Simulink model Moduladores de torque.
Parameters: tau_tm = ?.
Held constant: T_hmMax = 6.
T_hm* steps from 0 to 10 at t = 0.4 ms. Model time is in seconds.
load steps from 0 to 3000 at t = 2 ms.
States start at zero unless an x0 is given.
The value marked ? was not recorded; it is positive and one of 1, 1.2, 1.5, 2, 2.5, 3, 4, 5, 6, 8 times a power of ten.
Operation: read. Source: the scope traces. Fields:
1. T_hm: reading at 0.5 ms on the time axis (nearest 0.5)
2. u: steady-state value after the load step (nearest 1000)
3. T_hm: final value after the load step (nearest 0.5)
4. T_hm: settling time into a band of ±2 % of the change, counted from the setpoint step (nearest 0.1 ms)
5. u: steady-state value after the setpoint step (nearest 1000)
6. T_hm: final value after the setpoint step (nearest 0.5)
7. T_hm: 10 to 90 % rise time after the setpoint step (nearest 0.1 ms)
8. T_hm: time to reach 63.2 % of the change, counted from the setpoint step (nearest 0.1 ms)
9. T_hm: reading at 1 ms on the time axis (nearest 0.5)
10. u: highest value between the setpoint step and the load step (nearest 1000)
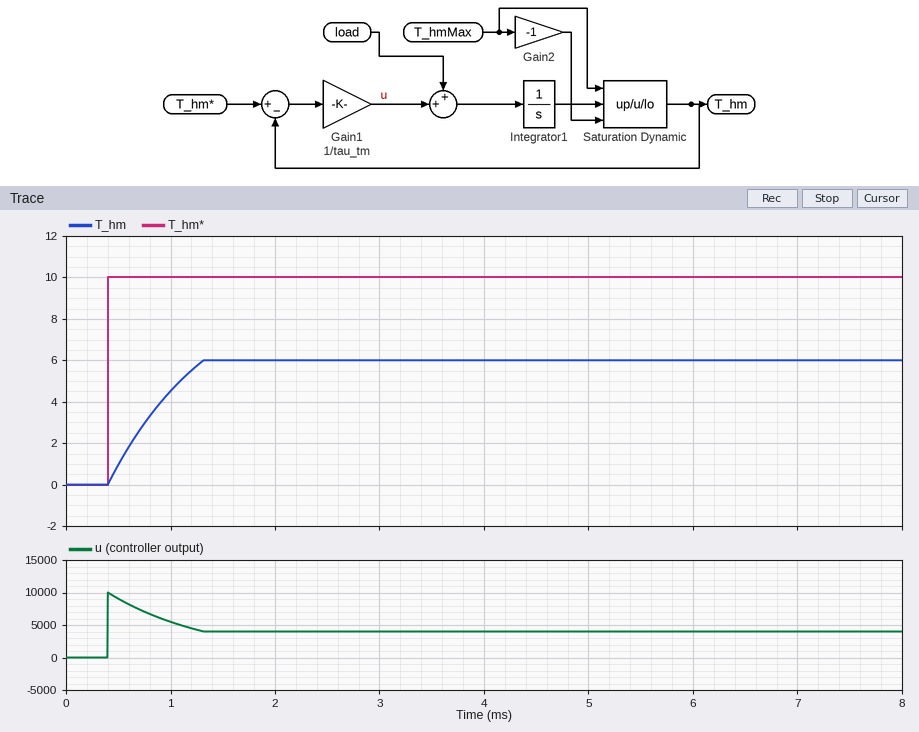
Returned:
1.0
4000
6.0
0.9 ms
4000
6.0
0.7 ms
0.5 ms
4.5
10000
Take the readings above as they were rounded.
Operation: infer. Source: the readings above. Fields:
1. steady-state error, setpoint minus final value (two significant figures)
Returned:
4.0
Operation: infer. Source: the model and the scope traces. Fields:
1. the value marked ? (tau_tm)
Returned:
0.001
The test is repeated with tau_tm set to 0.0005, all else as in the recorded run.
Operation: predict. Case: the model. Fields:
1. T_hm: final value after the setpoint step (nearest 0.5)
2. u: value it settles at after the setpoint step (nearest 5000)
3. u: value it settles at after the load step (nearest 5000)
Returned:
6.0
10000
10000
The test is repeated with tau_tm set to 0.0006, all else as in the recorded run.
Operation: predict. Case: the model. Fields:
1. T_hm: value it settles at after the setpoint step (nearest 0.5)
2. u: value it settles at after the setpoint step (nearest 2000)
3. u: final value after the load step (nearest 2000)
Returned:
6.0
6000
6000
